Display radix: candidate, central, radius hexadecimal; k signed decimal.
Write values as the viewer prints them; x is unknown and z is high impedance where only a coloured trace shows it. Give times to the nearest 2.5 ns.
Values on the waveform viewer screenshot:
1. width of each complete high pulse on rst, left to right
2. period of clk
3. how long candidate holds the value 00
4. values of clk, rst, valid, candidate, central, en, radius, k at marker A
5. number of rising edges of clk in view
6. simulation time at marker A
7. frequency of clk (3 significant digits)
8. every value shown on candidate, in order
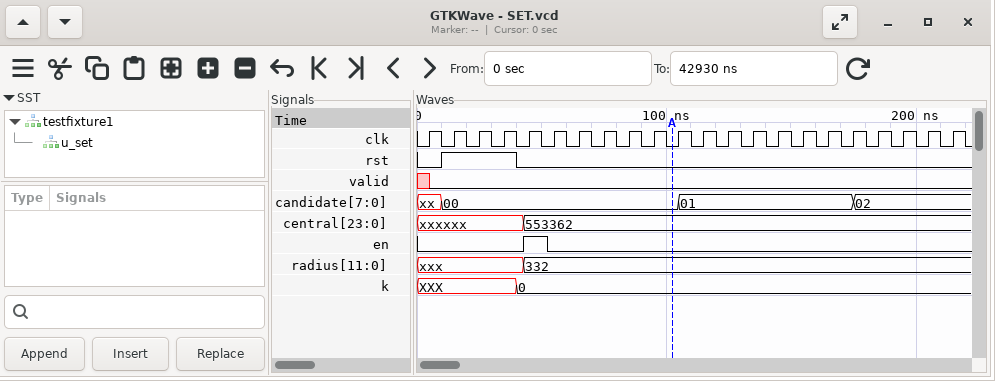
30 ns
10 ns
95 ns
clk=0, rst=0, valid=0, candidate=00, central=553362, en=0, radius=332, k=0
22
102.5 ns
100 MHz
xx, 00, 01, 02
